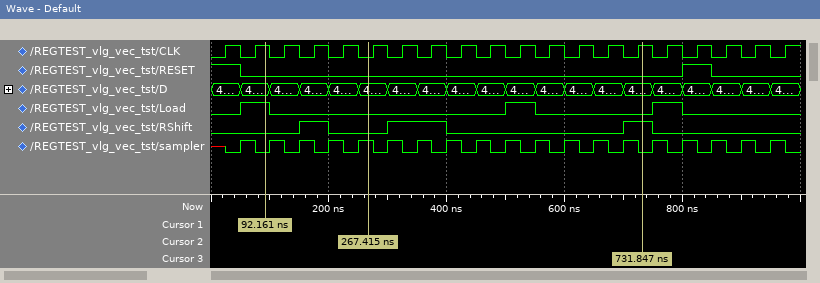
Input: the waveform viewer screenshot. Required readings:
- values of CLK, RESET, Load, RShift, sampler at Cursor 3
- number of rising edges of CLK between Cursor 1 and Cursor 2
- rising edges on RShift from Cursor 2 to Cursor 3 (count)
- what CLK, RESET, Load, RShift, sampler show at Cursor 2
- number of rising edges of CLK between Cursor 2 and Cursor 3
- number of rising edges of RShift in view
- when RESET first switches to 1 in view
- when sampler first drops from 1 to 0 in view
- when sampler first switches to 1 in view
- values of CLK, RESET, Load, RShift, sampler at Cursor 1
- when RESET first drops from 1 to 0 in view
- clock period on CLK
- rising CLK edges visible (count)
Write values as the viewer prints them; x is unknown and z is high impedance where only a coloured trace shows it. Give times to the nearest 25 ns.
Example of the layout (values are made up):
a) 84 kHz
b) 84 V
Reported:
a) CLK=1, RESET=0, Load=0, RShift=1, sampler=0
b) 3
c) 2
d) CLK=0, RESET=0, Load=0, RShift=0, sampler=1
e) 10
f) 3
g) 800 ns
h) 75 ns
i) 50 ns
j) CLK=1, RESET=0, Load=1, RShift=0, sampler=0
k) 50 ns
l) 50 ns
m) 20
